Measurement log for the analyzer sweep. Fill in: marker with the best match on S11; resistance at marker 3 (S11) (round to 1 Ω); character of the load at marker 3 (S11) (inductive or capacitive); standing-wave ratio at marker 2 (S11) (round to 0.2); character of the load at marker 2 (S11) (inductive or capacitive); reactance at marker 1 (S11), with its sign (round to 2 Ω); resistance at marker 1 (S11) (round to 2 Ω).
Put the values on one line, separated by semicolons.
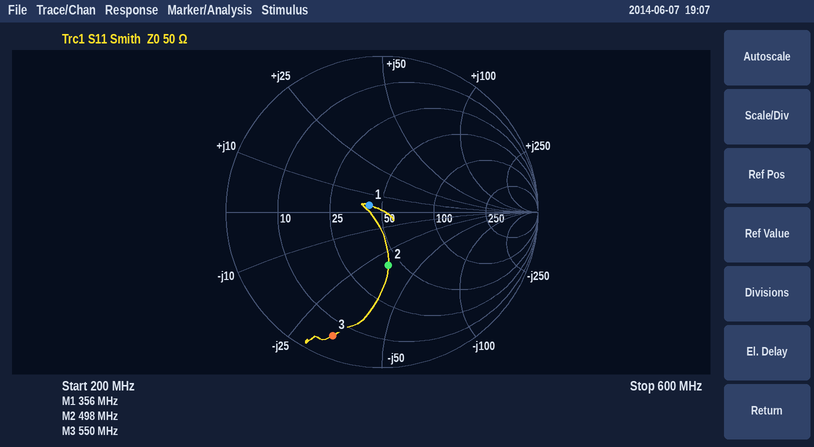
marker 1; 6 Ω; capacitive; 2.0; capacitive; +4 Ω; 42 Ω
